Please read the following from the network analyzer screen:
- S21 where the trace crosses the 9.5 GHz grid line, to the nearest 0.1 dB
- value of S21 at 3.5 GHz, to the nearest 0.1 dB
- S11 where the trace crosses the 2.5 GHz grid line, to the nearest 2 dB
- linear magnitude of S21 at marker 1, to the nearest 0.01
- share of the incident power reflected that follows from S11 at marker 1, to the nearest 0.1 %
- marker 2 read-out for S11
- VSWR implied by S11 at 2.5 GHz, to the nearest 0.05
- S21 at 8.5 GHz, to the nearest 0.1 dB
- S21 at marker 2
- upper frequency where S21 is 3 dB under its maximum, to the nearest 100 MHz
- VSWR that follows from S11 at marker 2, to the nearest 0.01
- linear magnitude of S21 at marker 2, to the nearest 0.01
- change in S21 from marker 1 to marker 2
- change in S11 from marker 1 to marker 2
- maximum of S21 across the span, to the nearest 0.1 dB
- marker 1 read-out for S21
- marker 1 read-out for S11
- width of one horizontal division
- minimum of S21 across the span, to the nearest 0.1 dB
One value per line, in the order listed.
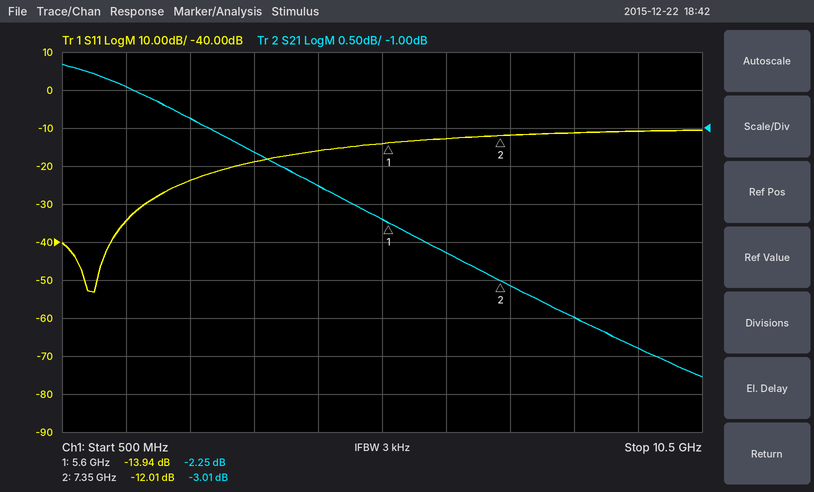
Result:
-3.9 dB
-1.3 dB
-24 dB
0.77
4.0 %
-12.01 dB
1.15
-3.5 dB
-3.01 dB
7.7 GHz
1.67
0.71
-0.76 dB
1.93 dB
-0.2 dB
-2.25 dB
-13.94 dB
1 GHz
-4.3 dB
